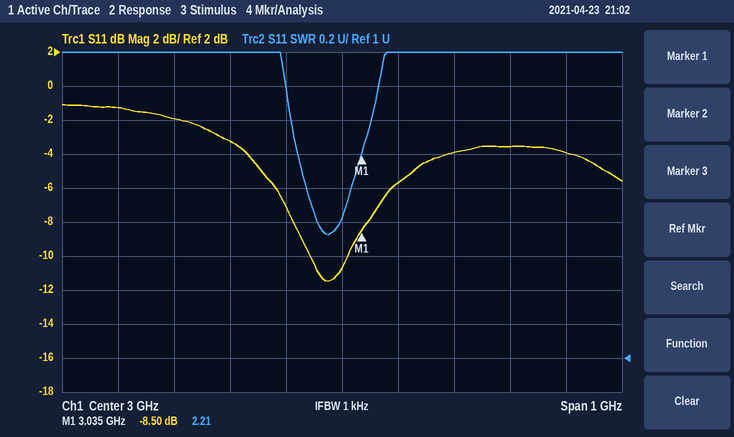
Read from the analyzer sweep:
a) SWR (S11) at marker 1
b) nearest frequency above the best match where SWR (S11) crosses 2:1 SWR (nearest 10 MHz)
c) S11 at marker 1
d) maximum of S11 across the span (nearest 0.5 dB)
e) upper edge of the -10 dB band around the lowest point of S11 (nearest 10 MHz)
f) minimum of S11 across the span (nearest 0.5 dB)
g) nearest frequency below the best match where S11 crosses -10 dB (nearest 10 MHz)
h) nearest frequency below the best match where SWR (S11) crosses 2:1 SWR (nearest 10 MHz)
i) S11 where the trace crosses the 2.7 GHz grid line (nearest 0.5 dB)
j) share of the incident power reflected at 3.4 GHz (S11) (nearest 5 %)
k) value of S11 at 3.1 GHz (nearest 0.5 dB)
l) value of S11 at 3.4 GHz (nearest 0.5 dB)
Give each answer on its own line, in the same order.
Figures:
2.21
3.02 GHz
-8.50 dB
-1.0 dB
3.01 GHz
-11.5 dB
2.94 GHz
2.94 GHz
-2.0 dB
40 %
-5.5 dB
-4.0 dB
